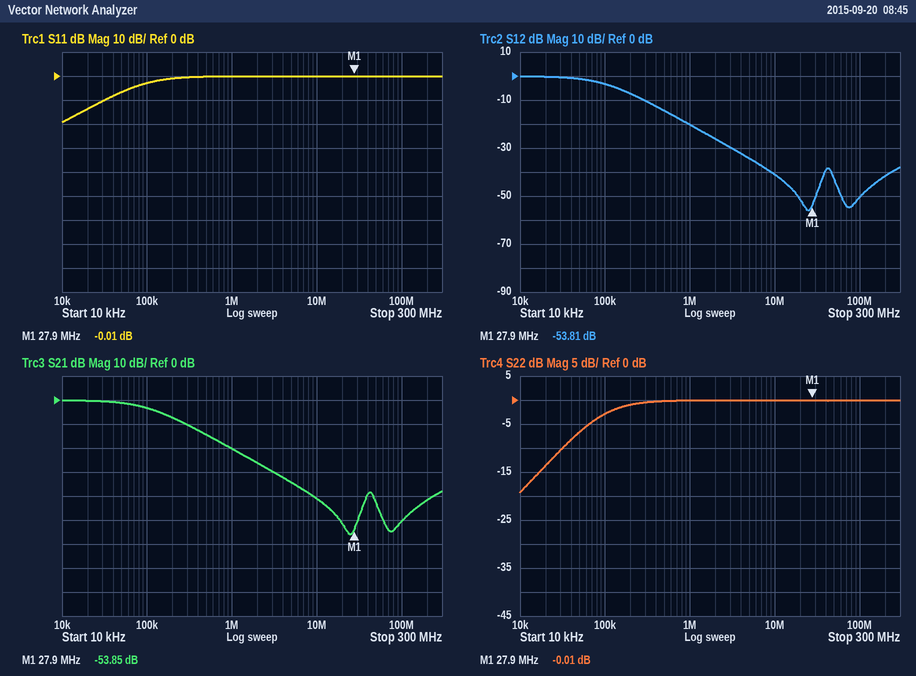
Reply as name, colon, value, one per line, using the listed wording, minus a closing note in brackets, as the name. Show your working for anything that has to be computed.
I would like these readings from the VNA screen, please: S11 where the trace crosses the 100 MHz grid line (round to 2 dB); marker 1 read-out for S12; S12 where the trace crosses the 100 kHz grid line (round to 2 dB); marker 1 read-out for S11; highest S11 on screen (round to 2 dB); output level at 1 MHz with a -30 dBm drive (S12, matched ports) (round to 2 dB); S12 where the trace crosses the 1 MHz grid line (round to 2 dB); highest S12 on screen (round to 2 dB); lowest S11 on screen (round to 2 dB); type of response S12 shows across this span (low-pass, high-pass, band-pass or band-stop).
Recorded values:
S11 where the trace crosses the 100 MHz grid line: 0 dB
marker 1 read-out for S12: -53.81 dB
S12 where the trace crosses the 100 kHz grid line: -4 dB
marker 1 read-out for S11: -0.01 dB
highest S11 on screen: 0 dB
output level at 1 MHz with a -30 dBm drive (S12, matched ports): -30 dBm + (-20 dB) = -50 dBm
S12 where the trace crosses the 1 MHz grid line: -20 dB
highest S12 on screen: 0 dB
lowest S11 on screen: -20 dB
type of response S12 shows across this span: low-pass
